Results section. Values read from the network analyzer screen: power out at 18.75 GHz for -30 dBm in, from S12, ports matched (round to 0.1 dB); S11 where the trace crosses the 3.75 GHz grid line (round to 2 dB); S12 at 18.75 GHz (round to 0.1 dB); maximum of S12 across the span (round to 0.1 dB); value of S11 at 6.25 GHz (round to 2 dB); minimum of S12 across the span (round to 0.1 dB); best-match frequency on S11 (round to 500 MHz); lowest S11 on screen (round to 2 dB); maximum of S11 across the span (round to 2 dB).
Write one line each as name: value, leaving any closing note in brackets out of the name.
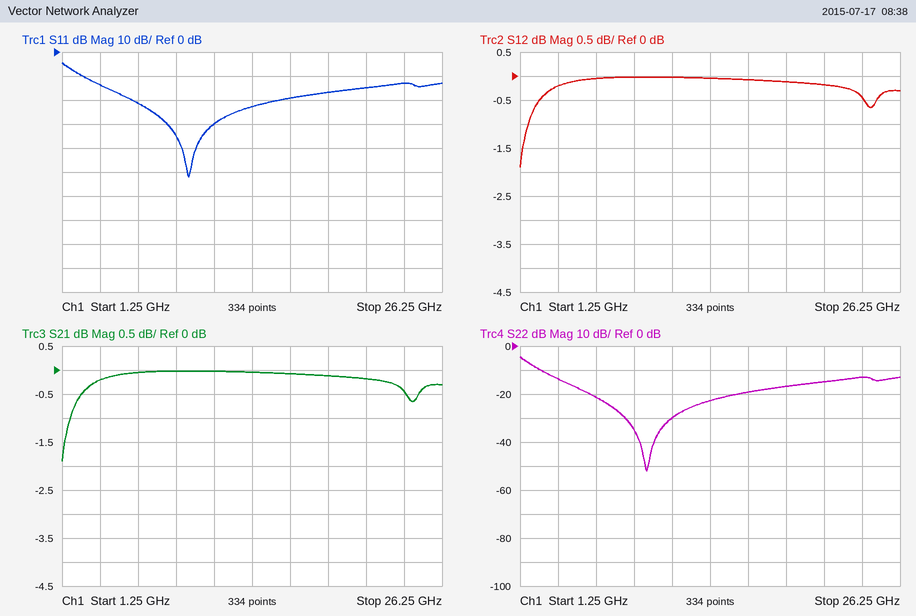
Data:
power out at 18.75 GHz for -30 dBm in, from S12, ports matched: -30.1 dBm
S11 where the trace crosses the 3.75 GHz grid line: -14 dB
S12 at 18.75 GHz: -0.1 dB
maximum of S12 across the span: 0.0 dB
value of S11 at 6.25 GHz: -22 dB
minimum of S12 across the span: -1.9 dB
best-match frequency on S11: 9.5 GHz
lowest S11 on screen: -52 dB
maximum of S11 across the span: -4 dB
